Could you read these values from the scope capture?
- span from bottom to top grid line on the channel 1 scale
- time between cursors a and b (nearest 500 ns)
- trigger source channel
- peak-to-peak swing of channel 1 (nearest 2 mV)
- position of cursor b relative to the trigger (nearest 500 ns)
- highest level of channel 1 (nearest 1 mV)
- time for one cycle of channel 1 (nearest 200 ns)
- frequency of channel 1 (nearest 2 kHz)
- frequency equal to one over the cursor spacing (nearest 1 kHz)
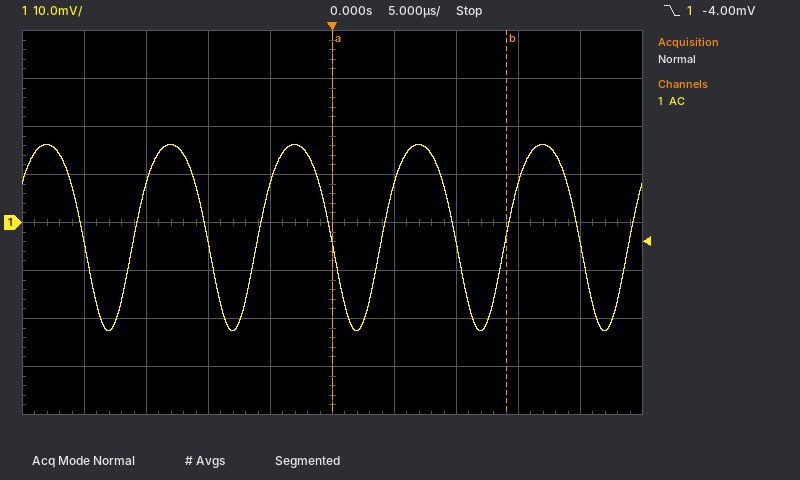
80 mV
14.0 µs
channel 1
38 mV
+14.0 µs
16 mV
10.0 µs
100 kHz
71 kHz
